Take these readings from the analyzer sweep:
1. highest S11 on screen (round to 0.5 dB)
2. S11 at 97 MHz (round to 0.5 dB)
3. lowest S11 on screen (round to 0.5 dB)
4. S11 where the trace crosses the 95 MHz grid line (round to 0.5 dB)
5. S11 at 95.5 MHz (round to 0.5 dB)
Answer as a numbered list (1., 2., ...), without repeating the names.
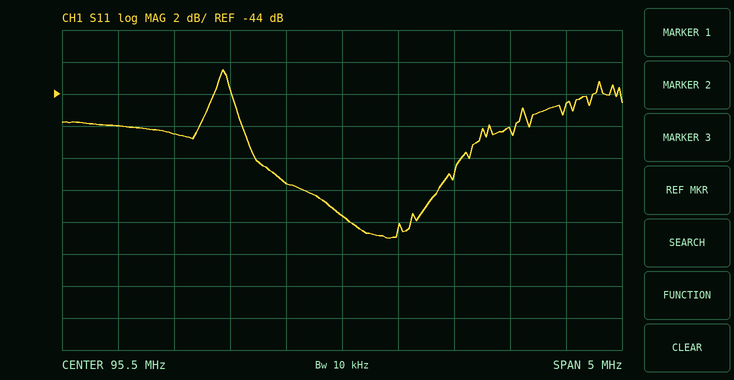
1. -42.5 dB
2. -46.0 dB
3. -53.0 dB
4. -49.5 dB
5. -51.5 dB
